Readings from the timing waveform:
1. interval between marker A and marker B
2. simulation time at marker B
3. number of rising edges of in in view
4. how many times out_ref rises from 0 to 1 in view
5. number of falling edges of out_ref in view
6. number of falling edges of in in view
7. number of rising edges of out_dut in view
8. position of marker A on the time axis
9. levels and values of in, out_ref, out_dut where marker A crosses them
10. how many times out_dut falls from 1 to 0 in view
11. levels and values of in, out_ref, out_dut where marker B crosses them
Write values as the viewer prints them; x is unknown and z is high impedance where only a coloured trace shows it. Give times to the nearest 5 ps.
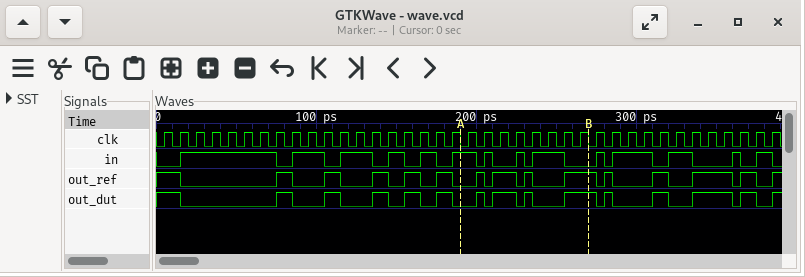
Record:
80 ps
270 ps
14
14
14
14
14
190 ps
in=1, out_ref=0, out_dut=0
14
in=0, out_ref=1, out_dut=1
